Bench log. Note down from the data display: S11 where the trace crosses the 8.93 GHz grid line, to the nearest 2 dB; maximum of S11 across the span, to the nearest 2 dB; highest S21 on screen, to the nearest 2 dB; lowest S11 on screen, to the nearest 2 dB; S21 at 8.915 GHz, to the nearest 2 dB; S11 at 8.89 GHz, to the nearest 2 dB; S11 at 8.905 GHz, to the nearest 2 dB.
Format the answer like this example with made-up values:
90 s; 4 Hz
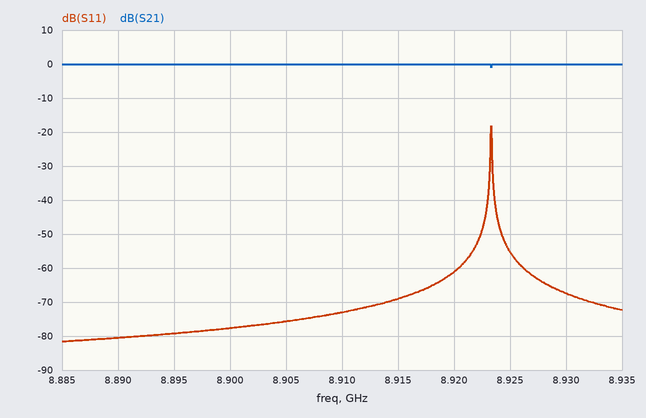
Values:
-68 dB; -18 dB; 0 dB; -82 dB; 0 dB; -80 dB; -76 dB
